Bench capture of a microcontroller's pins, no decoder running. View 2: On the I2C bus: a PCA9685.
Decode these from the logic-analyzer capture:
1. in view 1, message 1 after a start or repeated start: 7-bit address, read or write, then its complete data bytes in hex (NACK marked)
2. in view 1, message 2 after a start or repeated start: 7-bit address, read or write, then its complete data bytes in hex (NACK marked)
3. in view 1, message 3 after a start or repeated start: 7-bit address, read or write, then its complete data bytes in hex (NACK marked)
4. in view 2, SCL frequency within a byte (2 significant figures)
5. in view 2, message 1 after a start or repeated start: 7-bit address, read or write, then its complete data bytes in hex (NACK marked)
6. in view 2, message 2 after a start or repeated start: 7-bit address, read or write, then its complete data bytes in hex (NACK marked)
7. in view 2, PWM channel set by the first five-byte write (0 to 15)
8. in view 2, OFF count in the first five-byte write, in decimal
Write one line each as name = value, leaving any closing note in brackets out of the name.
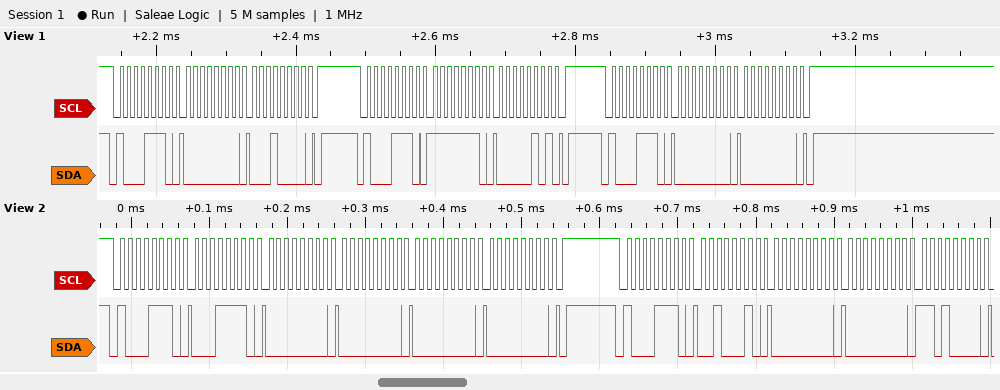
in view 1, message 1 after a start or repeated start: 7-bit address, read or write, then its complete data bytes in hex = 0x47 write: 00 10
in view 1, message 2 after a start or repeated start: 7-bit address, read or write, then its complete data bytes in hex = 0x47 write: FE 05
in view 1, message 3 after a start or repeated start: 7-bit address, read or write, then its complete data bytes in hex = 0x47 write: 00 00
in view 2, SCL frequency within a byte = 100 kHz
in view 2, message 1 after a start or repeated start: 7-bit address, read or write, then its complete data bytes in hex = 0x47 write: 1E 00 00 00 00
in view 2, message 2 after a start or repeated start: 7-bit address, read or write, then its complete data bytes in hex = 0x47 write: 22 00 00 D0
in view 2, PWM channel set by the first five-byte write = 6
in view 2, OFF count in the first five-byte write, in decimal = 0
